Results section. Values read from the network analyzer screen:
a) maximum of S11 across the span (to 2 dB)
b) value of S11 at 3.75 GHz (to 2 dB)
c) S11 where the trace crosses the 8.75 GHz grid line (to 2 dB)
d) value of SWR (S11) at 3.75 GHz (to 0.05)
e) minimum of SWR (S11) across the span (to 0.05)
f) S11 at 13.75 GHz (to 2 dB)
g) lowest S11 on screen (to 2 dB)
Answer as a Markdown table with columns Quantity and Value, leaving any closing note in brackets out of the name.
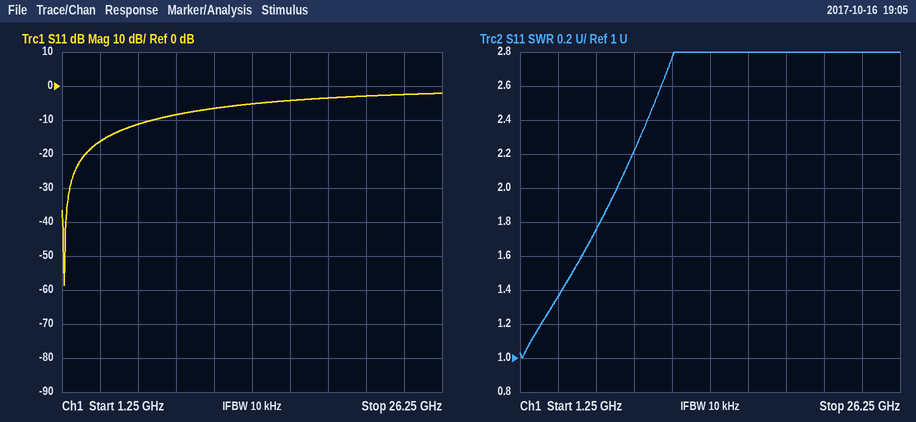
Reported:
| Quantity | Value |
|---|---|
| maximum of S11 across the span | -2 dB |
| value of S11 at 3.75 GHz | -16 dB |
| S11 where the trace crosses the 8.75 GHz grid line | -8 dB |
| value of SWR (S11) at 3.75 GHz | 1.35 |
| minimum of SWR (S11) across the span | 1.00 |
| S11 at 13.75 GHz | -6 dB |
| lowest S11 on screen | -58 dB |
